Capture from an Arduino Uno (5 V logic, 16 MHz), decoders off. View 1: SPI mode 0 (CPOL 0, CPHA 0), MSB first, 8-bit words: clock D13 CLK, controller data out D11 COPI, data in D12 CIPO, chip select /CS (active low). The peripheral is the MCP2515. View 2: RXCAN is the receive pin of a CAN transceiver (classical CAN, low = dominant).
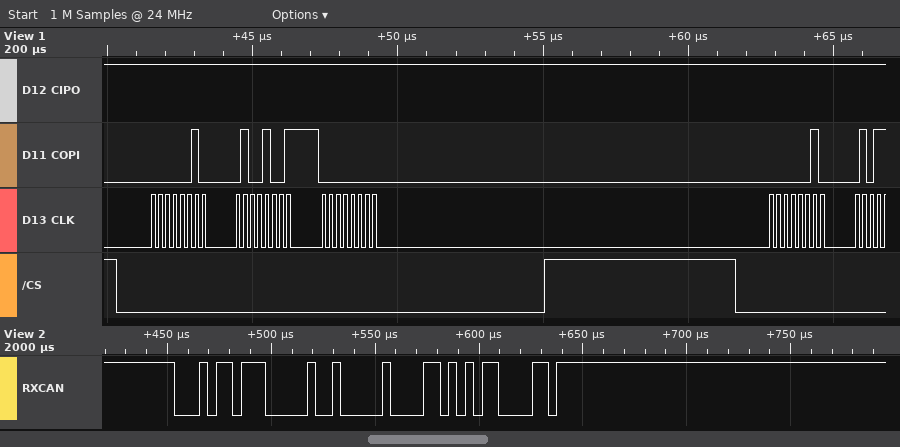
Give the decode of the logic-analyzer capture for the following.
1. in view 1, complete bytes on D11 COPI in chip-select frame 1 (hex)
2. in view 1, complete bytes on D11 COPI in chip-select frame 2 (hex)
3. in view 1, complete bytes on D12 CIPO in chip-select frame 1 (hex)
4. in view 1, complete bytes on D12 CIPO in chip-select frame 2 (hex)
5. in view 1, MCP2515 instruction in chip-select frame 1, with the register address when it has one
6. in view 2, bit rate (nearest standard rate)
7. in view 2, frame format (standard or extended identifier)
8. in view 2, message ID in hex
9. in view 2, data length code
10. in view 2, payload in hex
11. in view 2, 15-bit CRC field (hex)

02 49 00
02
FF FF FF
FF
WRITE 0x49
250 kbit/s
standard
0x16E
1
00
0x3561
